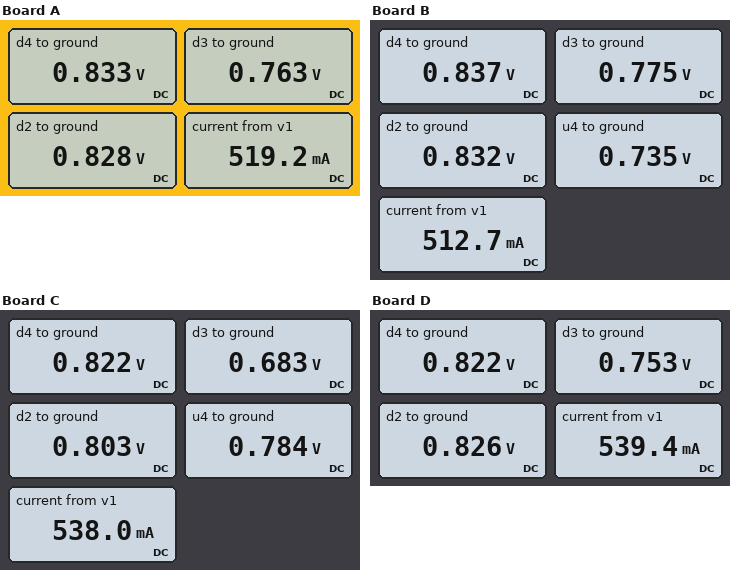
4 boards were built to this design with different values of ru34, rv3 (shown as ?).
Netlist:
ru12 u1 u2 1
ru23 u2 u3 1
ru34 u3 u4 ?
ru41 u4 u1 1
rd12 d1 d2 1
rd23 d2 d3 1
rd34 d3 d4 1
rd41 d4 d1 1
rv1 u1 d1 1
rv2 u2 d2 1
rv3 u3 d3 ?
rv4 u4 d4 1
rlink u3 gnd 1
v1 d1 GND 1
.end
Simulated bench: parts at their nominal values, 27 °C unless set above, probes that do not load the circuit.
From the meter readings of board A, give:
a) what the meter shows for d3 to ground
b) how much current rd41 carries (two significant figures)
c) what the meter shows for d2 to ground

0.763 V
170 mA
0.828 V
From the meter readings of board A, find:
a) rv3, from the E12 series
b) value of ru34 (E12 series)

1.8 Ω
1.2 Ω
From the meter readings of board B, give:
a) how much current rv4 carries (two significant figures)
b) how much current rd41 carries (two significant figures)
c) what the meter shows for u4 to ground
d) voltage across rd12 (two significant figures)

100 mA
160 mA
0.735 V
170 mV
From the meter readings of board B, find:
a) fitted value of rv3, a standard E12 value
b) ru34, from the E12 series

2.2 Ω
1.2 Ω
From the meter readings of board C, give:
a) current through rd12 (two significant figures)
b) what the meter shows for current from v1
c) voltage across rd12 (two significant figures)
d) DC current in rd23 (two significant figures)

200 mA
538.0 mA
200 mV
120 mA
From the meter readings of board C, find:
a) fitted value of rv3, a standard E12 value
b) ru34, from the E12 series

0.56 Ω
2.7 Ω
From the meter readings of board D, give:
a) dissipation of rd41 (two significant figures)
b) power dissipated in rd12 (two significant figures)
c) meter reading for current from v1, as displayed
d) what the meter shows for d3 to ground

32 mW
30 mW
539.4 mA
0.753 V
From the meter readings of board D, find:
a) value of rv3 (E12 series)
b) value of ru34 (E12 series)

1.5 Ω
0.82 Ω
